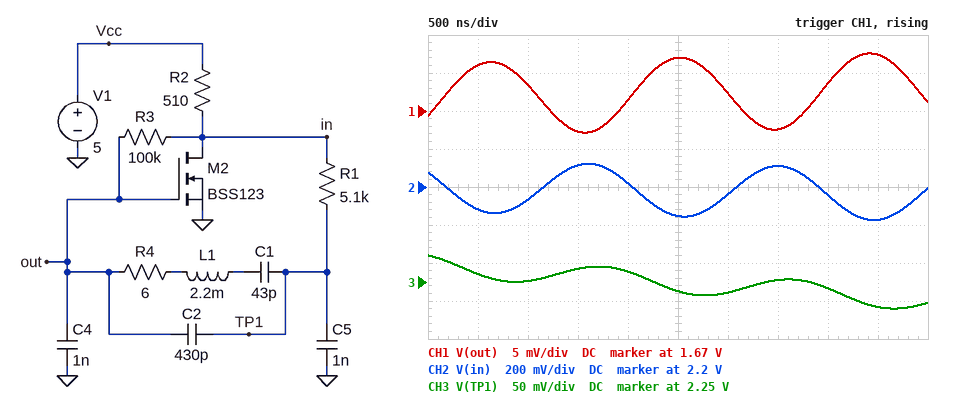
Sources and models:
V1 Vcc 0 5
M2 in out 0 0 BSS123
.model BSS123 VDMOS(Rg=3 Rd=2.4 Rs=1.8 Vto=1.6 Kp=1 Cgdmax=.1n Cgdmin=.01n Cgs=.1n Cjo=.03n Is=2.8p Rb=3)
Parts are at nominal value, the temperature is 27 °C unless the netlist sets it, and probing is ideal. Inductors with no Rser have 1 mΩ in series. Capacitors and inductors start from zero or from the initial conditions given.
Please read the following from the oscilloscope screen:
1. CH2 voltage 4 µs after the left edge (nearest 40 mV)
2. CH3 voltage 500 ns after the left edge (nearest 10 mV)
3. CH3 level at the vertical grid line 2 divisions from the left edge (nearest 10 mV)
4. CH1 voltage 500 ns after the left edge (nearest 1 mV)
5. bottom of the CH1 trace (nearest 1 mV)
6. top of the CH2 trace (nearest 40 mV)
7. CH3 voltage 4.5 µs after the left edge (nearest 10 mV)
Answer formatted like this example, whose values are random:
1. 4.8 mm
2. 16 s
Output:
1. 2.16 V
2. 2.26 V
3. 2.25 V
4. 1.676 V
5. 1.667 V
6. 2.32 V
7. 2.22 V
